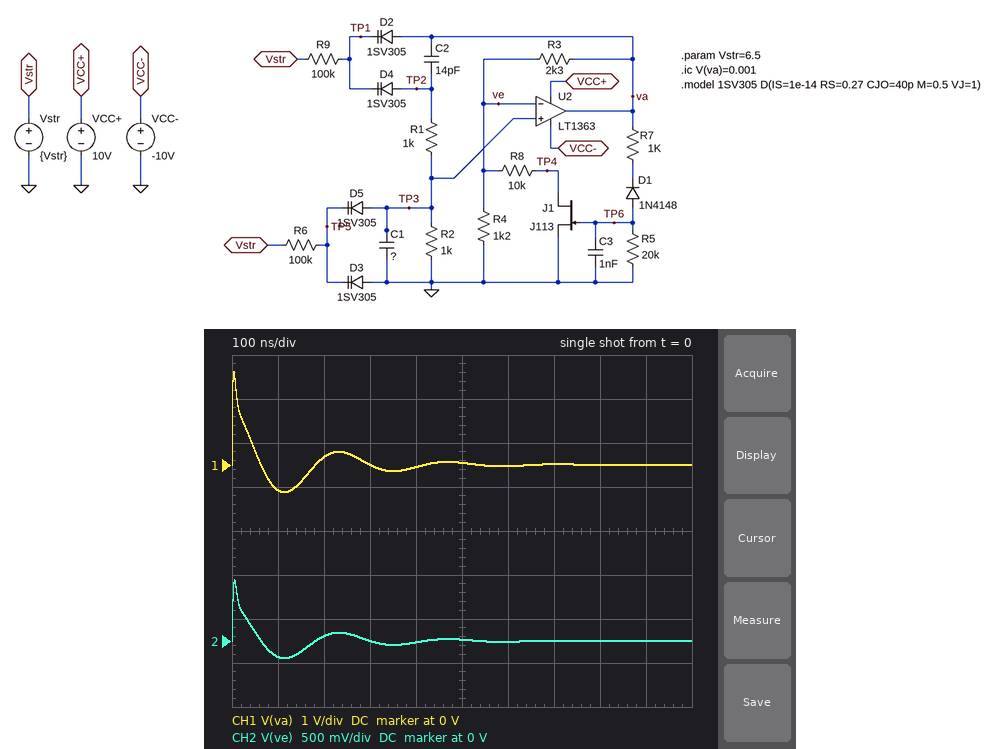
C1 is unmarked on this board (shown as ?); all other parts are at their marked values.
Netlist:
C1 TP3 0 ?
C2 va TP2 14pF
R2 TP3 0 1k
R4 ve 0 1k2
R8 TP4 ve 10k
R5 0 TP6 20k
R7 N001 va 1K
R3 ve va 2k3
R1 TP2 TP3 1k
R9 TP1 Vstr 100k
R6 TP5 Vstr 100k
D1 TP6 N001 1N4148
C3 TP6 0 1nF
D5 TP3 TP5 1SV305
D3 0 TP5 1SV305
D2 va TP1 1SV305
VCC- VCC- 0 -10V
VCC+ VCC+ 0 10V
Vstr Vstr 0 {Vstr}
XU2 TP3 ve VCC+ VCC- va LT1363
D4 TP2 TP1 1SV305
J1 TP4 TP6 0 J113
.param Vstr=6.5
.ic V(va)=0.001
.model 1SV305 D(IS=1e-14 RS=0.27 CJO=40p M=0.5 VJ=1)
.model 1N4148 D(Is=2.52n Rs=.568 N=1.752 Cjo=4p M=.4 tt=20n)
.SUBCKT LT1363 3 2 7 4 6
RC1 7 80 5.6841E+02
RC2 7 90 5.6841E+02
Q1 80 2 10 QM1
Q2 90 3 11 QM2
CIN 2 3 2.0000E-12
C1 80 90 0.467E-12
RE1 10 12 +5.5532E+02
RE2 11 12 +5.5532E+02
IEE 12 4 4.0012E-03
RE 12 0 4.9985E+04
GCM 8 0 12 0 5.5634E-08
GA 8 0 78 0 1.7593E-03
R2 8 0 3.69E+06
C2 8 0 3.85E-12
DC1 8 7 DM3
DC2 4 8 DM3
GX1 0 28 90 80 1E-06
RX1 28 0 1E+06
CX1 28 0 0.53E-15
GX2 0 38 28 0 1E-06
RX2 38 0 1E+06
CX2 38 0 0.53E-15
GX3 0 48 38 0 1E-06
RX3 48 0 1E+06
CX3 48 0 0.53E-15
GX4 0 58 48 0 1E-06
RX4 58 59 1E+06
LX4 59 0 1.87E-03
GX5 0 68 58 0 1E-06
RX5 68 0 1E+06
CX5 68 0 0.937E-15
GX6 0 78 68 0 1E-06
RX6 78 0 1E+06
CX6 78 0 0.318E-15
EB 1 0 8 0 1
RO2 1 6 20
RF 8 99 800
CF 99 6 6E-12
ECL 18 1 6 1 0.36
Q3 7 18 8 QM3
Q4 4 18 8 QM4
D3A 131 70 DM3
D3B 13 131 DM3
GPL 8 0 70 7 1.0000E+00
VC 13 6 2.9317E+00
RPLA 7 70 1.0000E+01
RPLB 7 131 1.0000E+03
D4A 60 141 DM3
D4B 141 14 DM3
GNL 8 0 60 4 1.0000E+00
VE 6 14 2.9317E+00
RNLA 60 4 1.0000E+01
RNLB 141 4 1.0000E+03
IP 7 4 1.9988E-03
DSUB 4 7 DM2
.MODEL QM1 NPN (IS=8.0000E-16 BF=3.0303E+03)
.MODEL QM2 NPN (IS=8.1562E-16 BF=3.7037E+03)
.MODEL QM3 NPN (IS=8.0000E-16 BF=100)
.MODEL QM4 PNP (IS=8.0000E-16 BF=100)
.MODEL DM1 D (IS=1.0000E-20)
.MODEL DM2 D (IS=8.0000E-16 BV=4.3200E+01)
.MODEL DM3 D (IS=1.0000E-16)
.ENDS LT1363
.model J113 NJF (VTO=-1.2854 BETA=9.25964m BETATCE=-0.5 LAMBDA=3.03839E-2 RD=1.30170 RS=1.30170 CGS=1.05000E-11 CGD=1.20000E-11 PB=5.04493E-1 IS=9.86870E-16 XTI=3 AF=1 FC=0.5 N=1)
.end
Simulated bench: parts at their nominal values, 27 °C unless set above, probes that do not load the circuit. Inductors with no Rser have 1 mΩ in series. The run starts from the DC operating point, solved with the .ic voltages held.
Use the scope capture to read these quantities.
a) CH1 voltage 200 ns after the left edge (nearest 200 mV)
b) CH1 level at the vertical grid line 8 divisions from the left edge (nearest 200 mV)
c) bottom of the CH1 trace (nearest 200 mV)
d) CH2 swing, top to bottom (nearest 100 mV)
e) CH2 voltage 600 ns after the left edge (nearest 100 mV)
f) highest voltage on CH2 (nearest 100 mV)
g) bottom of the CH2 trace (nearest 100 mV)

200 mV
0 V
-600 mV
900 mV
0 V
700 mV
-200 mV
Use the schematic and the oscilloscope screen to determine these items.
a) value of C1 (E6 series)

33 pF
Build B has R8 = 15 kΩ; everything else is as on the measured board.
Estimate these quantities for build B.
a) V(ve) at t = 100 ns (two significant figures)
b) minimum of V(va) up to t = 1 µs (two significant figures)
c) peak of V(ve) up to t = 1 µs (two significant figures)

-180 mV
-570 mV
700 mV
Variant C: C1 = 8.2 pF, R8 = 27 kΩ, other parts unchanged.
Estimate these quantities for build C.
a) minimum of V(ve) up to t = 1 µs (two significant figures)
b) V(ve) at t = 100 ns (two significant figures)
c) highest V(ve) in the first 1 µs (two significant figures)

-2.9 V
-780 mV
2.9 V
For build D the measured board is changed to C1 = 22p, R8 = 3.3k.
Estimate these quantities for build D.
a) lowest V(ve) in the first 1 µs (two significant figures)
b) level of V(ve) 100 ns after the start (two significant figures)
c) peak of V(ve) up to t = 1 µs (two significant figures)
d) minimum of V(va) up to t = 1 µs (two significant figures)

-1.1 V
-360 mV
1.1 V
-4.0 V
